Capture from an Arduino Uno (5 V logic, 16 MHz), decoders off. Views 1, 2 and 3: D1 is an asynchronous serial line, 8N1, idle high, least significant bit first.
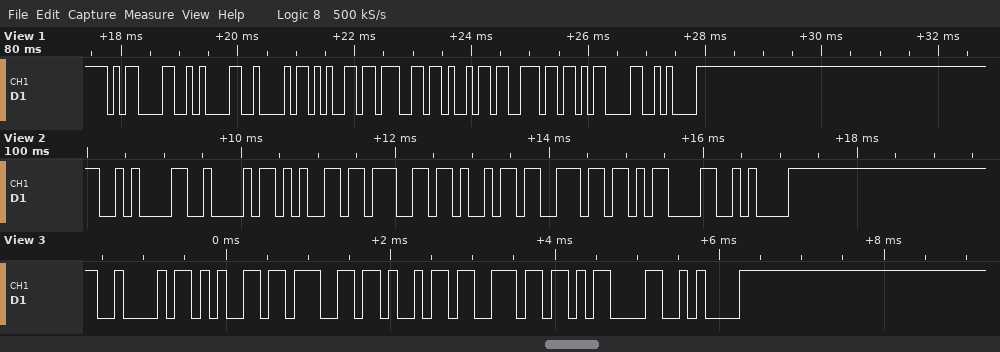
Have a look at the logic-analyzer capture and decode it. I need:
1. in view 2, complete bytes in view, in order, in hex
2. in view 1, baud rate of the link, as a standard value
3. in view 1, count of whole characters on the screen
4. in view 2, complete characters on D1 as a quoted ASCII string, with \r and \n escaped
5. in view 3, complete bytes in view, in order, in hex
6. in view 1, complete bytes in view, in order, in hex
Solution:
0A 42 65 67 69 6E 0D 0A
9600 baud
9
"\nBegin\r\n"
42 65 67 69 6E 0D 0A
0D 0A 42 65 67 69 6E 0D 0A
